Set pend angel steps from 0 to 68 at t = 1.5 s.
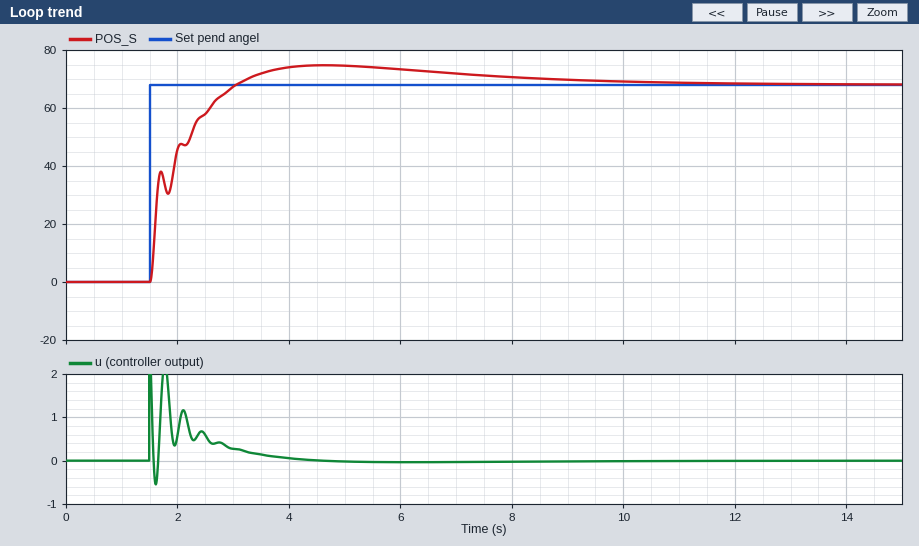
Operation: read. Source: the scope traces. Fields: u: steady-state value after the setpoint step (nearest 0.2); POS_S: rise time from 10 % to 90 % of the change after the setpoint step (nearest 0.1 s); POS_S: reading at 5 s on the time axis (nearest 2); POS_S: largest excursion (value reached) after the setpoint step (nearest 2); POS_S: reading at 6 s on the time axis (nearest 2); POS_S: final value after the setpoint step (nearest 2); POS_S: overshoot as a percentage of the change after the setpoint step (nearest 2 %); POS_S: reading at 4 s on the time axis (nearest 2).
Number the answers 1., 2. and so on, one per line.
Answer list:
1. 0.0
2. 1.1 s
3. 74
4. 74
5. 74
6. 68
7. 10 %
8. 74
